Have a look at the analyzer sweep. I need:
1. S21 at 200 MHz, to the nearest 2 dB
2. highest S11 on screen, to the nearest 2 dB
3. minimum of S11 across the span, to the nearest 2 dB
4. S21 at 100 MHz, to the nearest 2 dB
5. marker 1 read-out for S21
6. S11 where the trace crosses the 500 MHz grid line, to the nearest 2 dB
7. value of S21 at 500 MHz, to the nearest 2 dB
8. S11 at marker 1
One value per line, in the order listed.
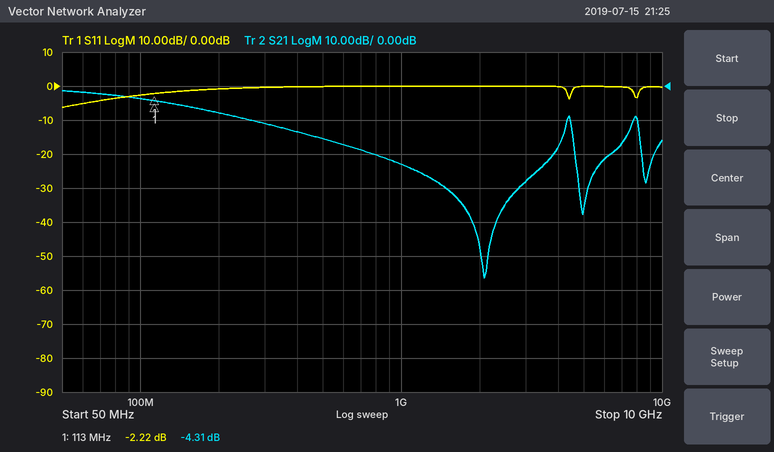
-8 dB
0 dB
-6 dB
-4 dB
-4.31 dB
0 dB
-16 dB
-2.22 dB
